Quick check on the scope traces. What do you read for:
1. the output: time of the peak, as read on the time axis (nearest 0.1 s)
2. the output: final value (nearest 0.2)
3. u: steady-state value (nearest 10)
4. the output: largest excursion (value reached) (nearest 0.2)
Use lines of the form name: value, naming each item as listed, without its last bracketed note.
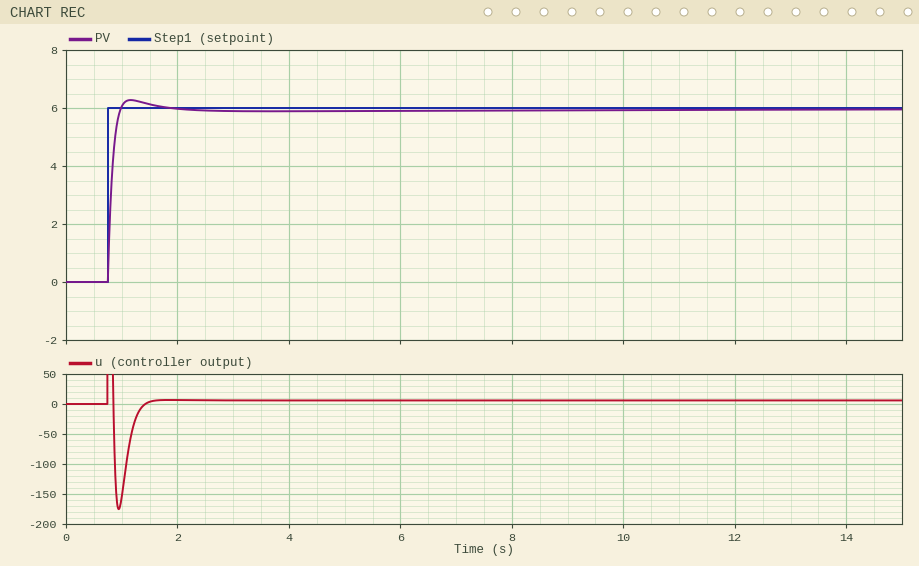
the output: time of the peak, as read on the time axis: 1.2 s
the output: final value: 6.0
u: steady-state value: 10
the output: largest excursion (value reached): 6.2
